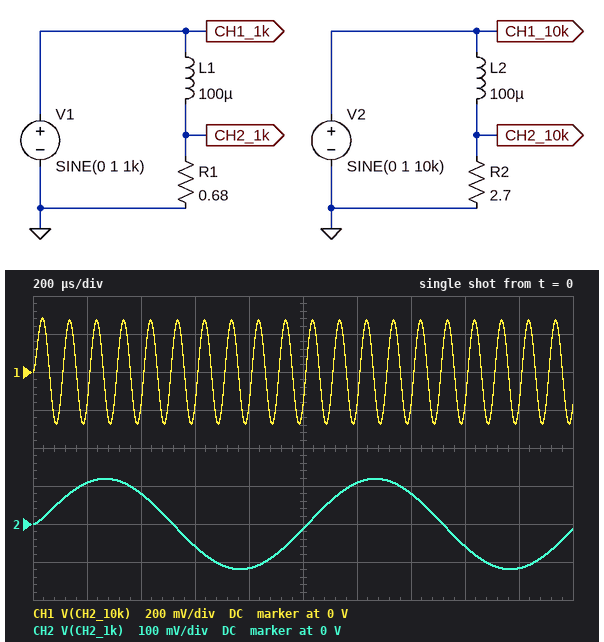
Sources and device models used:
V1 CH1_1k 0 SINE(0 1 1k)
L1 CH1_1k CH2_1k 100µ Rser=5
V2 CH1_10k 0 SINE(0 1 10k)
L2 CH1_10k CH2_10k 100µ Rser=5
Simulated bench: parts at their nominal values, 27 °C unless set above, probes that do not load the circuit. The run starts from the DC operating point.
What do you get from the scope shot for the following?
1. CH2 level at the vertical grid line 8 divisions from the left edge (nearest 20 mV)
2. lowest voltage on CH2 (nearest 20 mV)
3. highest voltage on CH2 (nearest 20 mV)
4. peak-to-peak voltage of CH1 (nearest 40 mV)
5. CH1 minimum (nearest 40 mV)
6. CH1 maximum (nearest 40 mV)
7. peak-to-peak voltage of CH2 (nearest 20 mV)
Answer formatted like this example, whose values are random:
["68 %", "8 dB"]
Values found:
["-60 mV", "-120 mV", "120 mV", "560 mV", "-280 mV", "280 mV", "240 mV"]
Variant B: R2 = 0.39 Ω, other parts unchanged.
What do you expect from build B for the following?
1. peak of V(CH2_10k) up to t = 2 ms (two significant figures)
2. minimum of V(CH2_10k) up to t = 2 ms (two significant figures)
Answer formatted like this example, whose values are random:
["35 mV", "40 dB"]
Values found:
["52 mV", "-47 mV"]
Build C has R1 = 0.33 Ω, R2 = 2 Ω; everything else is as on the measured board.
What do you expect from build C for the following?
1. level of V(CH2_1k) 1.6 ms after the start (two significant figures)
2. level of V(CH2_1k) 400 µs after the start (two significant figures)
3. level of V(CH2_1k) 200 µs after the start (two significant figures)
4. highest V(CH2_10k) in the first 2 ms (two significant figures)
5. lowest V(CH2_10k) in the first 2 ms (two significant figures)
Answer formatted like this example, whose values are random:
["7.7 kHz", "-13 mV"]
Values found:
["-30 mV", "42 mV", "56 mV", "220 mV", "-210 mV"]
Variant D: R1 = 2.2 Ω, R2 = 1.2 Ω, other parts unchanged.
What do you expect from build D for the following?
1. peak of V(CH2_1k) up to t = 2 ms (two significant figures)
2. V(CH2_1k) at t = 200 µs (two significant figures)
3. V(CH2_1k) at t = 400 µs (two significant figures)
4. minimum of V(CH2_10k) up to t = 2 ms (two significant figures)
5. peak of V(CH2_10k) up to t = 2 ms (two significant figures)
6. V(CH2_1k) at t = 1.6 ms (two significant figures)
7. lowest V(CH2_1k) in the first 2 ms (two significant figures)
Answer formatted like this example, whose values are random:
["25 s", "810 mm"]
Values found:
["300 mV", "280 mV", "200 mV", "-140 mV", "150 mV", "-160 mV", "-300 mV"]
